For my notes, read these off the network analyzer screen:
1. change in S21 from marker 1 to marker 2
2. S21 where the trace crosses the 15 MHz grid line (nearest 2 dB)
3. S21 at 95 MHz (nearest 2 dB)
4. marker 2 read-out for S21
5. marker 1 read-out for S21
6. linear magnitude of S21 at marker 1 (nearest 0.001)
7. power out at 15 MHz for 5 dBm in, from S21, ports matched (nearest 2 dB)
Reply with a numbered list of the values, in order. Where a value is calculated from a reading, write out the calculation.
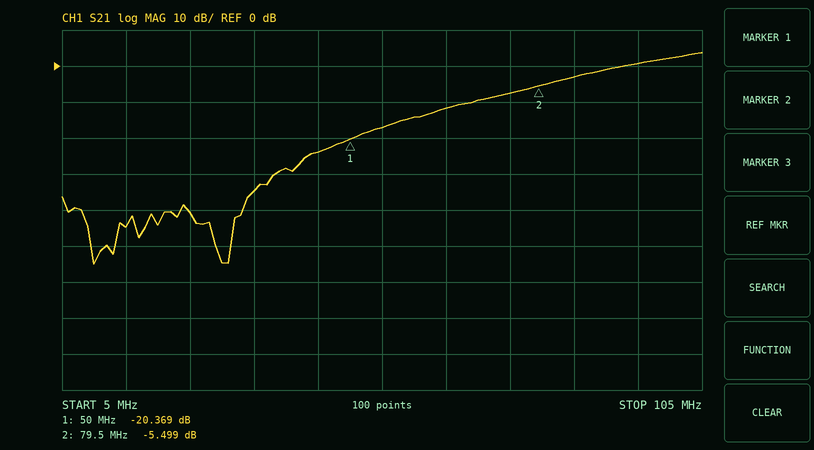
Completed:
1. -5.499 − (-20.369) = 14.870 dB
2. -44 dB
3. 0 dB
4. -5.499 dB
5. -20.369 dB
6. 10^(-20.369/20) ≈ 0.096
7. 5 dBm + (-44 dB) = -40 dBm
